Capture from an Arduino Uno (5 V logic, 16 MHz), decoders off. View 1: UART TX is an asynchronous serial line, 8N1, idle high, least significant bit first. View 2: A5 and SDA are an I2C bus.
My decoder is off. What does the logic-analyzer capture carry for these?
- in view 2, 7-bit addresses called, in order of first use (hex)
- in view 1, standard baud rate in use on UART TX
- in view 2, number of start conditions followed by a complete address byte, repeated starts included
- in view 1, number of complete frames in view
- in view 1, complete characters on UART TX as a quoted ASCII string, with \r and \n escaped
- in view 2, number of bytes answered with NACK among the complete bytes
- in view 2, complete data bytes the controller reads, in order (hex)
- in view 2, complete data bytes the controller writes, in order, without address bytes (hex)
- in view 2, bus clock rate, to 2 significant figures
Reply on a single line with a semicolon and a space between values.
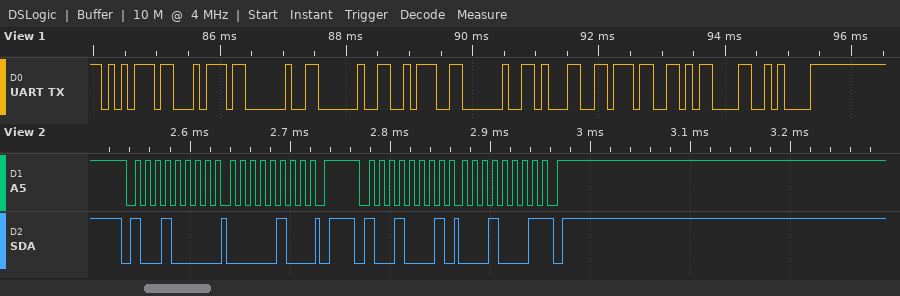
0x48; 9600 baud; 2; 10; "ut  : 17\r\n"; 1; 11; 04; 100 kHz
